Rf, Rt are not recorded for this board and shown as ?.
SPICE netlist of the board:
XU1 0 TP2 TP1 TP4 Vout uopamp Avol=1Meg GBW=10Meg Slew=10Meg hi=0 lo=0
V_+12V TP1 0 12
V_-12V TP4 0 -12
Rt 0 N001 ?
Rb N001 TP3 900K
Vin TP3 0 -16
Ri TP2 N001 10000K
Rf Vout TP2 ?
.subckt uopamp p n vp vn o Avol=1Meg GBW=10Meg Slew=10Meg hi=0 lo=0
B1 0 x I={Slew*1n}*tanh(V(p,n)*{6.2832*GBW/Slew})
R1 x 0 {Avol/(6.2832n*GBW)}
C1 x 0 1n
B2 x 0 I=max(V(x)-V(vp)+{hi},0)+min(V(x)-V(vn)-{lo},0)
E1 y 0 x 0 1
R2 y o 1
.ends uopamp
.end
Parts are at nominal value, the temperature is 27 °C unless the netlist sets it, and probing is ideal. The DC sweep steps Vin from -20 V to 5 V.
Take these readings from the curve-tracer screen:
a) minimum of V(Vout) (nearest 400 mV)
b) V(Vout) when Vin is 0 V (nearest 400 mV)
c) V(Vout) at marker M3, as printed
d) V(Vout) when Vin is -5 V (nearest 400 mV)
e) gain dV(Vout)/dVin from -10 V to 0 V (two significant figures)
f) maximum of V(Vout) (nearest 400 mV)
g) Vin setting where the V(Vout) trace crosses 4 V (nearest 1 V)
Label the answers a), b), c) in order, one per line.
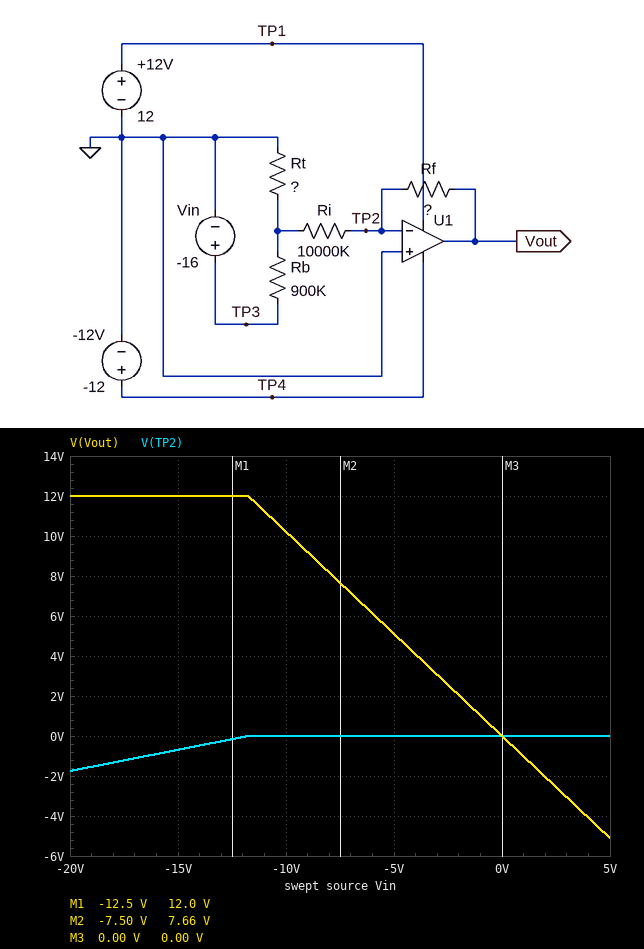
a) -5.2 V
b) 0 V
c) 0.00 V
d) 5.2 V
e) -1.0 V/V
f) 12.0 V
g) -4 V
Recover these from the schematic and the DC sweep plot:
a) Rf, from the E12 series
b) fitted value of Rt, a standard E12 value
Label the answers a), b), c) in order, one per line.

a) 39 MΩ
b) 330 kΩ
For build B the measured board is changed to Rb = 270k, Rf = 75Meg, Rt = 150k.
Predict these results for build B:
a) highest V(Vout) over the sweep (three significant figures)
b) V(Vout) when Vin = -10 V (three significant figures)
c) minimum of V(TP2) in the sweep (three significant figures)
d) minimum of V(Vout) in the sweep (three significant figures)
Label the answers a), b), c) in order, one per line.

a) 12.0 V
b) 12.0 V
c) -4.87 V
d) -12.0 V
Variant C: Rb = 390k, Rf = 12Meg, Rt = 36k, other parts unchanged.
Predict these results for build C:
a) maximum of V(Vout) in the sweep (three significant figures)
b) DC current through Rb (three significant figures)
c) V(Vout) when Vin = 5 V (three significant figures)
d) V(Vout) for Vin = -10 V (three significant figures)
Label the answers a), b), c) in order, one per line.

a) 2.02 V
b) 37.6 µA
c) -505 mV
d) 1.01 V
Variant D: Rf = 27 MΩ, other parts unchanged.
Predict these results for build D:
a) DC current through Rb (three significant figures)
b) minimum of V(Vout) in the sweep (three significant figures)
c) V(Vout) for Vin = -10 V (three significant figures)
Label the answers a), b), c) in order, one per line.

a) 13.1 µA
b) -3.54 V
c) 7.07 V
